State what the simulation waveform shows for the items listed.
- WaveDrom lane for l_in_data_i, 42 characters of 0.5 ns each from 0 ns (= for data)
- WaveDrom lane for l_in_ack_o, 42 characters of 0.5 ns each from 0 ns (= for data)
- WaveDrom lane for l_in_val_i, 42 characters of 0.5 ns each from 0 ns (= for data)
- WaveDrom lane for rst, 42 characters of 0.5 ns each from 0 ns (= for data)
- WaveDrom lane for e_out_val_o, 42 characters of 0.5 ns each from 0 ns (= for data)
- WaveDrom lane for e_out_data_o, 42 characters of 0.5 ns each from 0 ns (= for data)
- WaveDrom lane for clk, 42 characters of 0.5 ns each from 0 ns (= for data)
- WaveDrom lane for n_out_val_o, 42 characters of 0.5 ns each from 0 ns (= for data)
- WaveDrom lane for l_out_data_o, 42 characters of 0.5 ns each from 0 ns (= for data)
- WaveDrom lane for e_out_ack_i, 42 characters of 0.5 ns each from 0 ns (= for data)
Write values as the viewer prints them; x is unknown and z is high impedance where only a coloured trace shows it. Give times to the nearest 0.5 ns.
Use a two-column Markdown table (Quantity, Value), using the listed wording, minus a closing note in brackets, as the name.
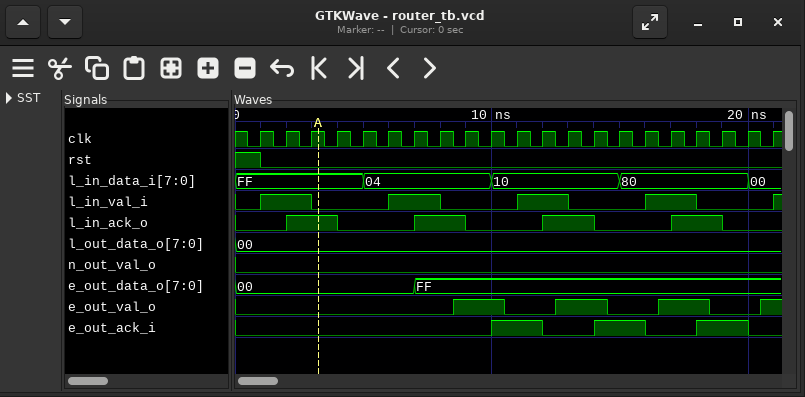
| Quantity | Value |
|---|---|
| WaveDrom lane for l_in_data_i, 42 characters of 0.5 ns each from 0 ns | {name: 'l_in_data_i', wave: '=.........=.........=.........=.........=.', data: 'FF 04 10 80 00'} |
| WaveDrom lane for l_in_ack_o, 42 characters of 0.5 ns each from 0 ns | {name: 'l_in_ack_o', wave: '0...1...0.....1...0.....1...0.....1...0...'} |
| WaveDrom lane for l_in_val_i, 42 characters of 0.5 ns each from 0 ns | {name: 'l_in_val_i', wave: '0.1...0.....1...0.....1...0.....1...0.....'} |
| WaveDrom lane for rst, 42 characters of 0.5 ns each from 0 ns | {name: 'rst', wave: '1.0.......................................'} |
| WaveDrom lane for e_out_val_o, 42 characters of 0.5 ns each from 0 ns | {name: 'e_out_val_o', wave: '0................1...0...1...0...1...0...1'} |
| WaveDrom lane for e_out_data_o, 42 characters of 0.5 ns each from 0 ns | {name: 'e_out_data_o', wave: '=.............=...........................', data: '00 FF'} |
| WaveDrom lane for clk, 42 characters of 0.5 ns each from 0 ns | {name: 'clk', wave: '101010101010101010101010101010101010101010'} |
| WaveDrom lane for n_out_val_o, 42 characters of 0.5 ns each from 0 ns | {name: 'n_out_val_o', wave: '0.........................................'} |
| WaveDrom lane for l_out_data_o, 42 characters of 0.5 ns each from 0 ns | {name: 'l_out_data_o', wave: '=.........................................', data: '00'} |
| WaveDrom lane for e_out_ack_i, 42 characters of 0.5 ns each from 0 ns | {name: 'e_out_ack_i', wave: '0...................1...0...1...0...1...0.'} |
